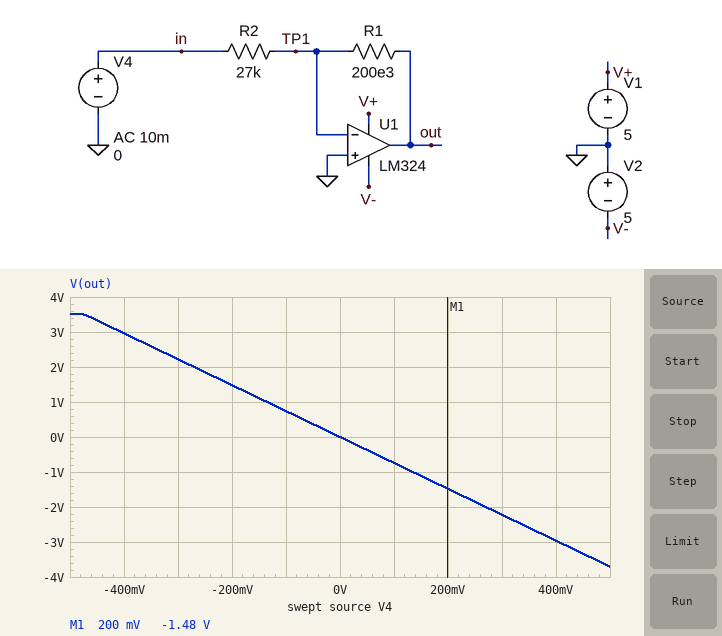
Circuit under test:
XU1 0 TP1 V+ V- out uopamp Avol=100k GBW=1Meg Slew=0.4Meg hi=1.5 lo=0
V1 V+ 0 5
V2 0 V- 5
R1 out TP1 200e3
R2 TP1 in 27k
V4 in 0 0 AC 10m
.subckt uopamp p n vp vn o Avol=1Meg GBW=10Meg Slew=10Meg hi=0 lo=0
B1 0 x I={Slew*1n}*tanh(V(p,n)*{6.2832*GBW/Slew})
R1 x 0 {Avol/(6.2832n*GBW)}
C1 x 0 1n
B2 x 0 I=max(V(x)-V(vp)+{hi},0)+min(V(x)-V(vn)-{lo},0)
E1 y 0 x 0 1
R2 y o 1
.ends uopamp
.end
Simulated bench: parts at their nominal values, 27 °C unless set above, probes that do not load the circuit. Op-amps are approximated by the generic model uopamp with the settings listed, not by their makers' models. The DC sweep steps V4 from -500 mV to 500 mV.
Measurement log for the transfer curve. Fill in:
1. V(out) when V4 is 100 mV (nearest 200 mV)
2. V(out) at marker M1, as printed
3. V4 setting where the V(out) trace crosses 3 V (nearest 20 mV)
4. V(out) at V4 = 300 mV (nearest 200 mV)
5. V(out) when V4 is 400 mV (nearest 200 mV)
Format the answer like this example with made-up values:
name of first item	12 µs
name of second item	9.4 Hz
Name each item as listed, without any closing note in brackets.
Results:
V(out) when V4 is 100 mV	-800 mV
V(out) at marker M1, as printed	-1.48 V
V4 setting where the V(out) trace crosses 3 V	-400 mV
V(out) at V4 = 300 mV	-2.2 V
V(out) when V4 is 400 mV	-3.0 V
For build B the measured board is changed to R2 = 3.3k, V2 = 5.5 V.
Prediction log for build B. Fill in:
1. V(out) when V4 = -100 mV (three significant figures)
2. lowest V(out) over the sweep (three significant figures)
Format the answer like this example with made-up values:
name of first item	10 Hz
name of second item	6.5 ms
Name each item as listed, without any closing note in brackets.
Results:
V(out) when V4 = -100 mV	3.50 V
lowest V(out) over the sweep	-5.50 V
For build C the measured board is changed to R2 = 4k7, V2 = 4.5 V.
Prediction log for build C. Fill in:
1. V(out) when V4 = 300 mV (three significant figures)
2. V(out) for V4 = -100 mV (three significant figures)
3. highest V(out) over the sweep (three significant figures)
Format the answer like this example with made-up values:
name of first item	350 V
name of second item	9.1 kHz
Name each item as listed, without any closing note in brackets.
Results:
V(out) when V4 = 300 mV	-4.50 V
V(out) for V4 = -100 mV	3.50 V
highest V(out) over the sweep	3.50 V
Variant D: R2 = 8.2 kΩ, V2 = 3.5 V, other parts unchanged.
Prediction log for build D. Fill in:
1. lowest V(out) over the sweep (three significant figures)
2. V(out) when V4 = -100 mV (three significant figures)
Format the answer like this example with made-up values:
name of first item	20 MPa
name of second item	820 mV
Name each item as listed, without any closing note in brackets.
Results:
lowest V(out) over the sweep	-3.50 V
V(out) when V4 = -100 mV	2.44 V
